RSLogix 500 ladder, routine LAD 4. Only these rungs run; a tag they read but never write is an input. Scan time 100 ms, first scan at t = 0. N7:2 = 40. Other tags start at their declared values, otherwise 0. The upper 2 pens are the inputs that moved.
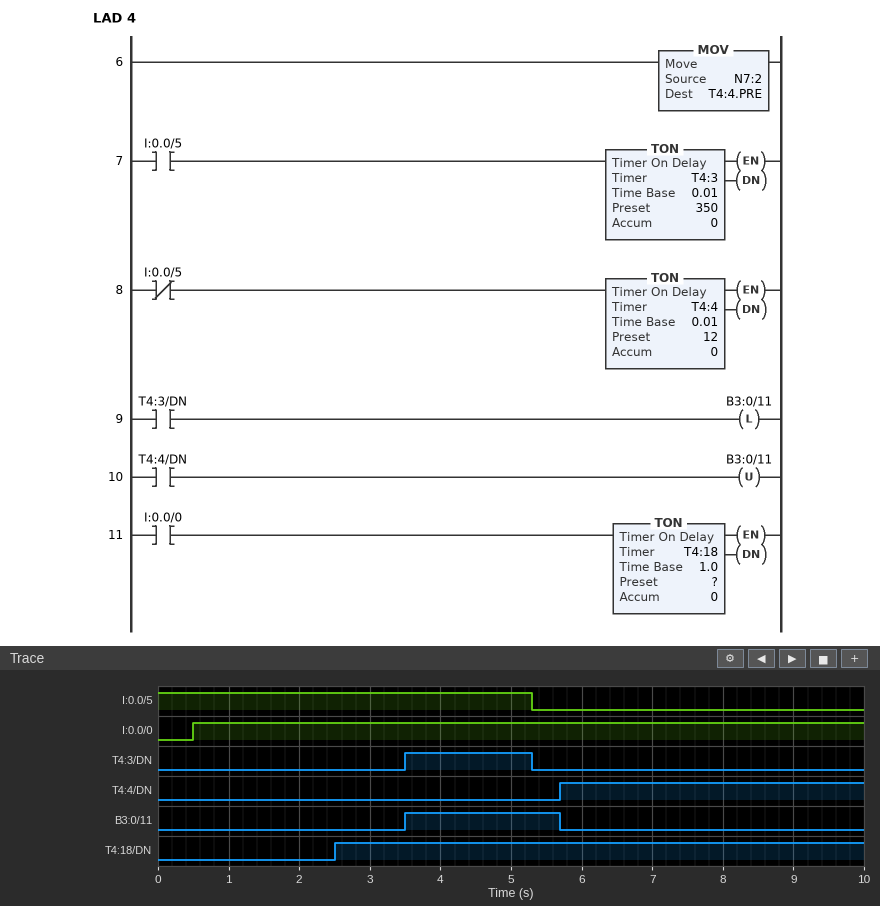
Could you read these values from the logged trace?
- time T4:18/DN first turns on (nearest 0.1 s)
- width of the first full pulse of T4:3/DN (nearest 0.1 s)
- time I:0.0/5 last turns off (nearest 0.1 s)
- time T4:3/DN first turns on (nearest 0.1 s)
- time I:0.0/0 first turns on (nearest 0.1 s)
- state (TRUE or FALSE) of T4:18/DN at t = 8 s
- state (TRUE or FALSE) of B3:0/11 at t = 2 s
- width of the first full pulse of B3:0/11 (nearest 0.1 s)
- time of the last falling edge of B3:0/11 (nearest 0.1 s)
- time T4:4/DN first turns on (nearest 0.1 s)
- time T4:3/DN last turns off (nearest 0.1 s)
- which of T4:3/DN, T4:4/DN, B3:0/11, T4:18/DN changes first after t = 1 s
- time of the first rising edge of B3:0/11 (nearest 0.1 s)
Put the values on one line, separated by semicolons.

2.5 s; 1.8 s; 5.3 s; 3.5 s; 0.5 s; TRUE; FALSE; 2.2 s; 5.7 s; 5.7 s; 5.3 s; T4:18/DN; 3.5 s
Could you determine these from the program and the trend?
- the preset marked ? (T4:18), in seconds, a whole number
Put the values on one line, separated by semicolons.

2 s
